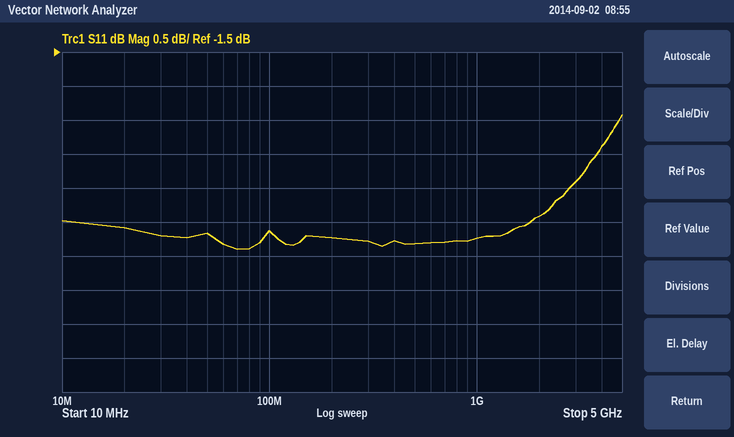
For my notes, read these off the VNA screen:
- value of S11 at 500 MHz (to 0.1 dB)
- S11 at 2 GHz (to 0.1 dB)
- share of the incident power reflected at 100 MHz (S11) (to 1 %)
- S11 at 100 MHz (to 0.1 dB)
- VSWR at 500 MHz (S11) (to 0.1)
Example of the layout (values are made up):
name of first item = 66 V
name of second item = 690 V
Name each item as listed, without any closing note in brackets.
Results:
value of S11 at 500 MHz = -4.3 dB
S11 at 2 GHz = -3.9 dB
share of the incident power reflected at 100 MHz (S11) = 39 %
S11 at 100 MHz = -4.1 dB
VSWR at 500 MHz (S11) = 4.1
